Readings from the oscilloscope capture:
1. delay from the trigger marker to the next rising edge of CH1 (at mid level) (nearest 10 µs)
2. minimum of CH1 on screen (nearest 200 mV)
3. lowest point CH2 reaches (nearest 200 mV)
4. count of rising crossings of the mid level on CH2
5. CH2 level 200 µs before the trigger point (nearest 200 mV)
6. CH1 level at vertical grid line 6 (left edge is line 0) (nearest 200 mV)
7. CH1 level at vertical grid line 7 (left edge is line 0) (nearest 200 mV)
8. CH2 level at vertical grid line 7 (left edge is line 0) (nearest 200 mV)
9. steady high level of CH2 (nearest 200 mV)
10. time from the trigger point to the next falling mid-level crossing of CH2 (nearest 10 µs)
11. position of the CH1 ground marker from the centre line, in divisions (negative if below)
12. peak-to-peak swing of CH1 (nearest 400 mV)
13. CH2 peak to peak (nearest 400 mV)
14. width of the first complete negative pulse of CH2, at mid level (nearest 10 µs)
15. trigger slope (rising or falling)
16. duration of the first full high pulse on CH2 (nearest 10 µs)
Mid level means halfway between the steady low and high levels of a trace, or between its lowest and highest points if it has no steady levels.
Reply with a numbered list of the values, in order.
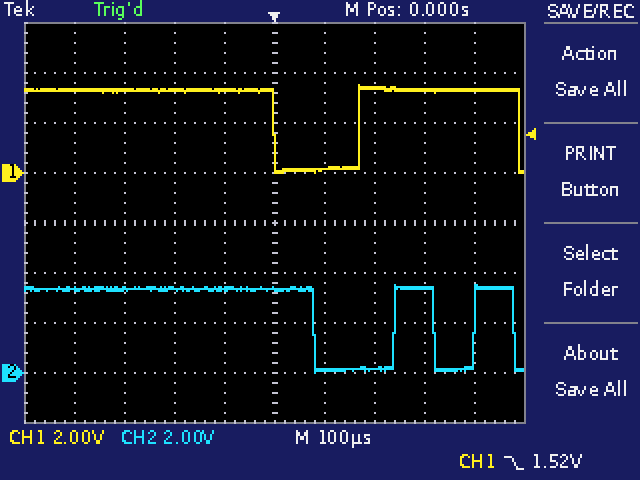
1. 170 µs
2. 0.0 V
3. 0.0 V
4. 2
5. 3.4 V
6. 200 mV
7. 3.4 V
8. 200 mV
9. 3.4 V
10. 80 µs
11. +1.0 div
12. 3.6 V
13. 3.6 V
14. 160 µs
15. falling
16. 80 µs
